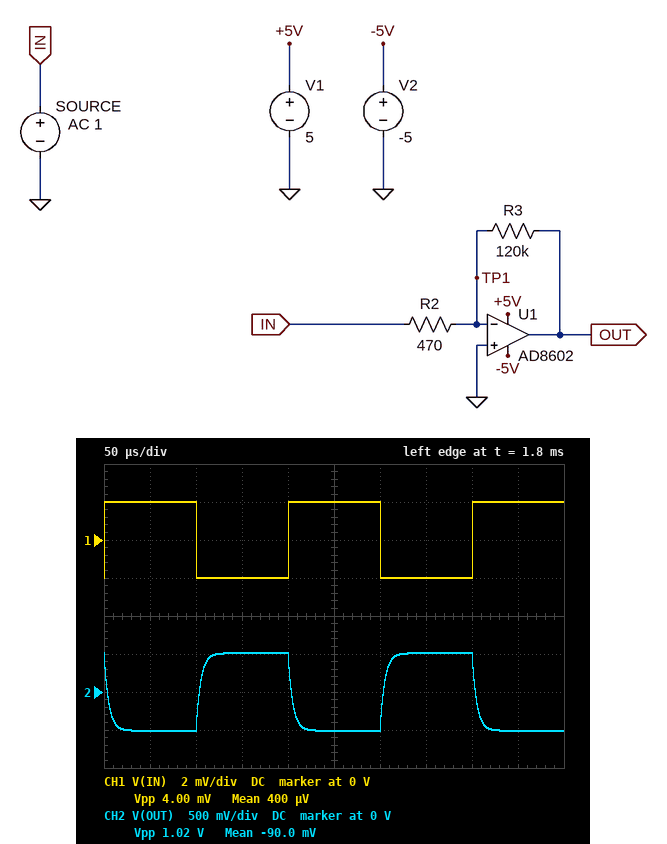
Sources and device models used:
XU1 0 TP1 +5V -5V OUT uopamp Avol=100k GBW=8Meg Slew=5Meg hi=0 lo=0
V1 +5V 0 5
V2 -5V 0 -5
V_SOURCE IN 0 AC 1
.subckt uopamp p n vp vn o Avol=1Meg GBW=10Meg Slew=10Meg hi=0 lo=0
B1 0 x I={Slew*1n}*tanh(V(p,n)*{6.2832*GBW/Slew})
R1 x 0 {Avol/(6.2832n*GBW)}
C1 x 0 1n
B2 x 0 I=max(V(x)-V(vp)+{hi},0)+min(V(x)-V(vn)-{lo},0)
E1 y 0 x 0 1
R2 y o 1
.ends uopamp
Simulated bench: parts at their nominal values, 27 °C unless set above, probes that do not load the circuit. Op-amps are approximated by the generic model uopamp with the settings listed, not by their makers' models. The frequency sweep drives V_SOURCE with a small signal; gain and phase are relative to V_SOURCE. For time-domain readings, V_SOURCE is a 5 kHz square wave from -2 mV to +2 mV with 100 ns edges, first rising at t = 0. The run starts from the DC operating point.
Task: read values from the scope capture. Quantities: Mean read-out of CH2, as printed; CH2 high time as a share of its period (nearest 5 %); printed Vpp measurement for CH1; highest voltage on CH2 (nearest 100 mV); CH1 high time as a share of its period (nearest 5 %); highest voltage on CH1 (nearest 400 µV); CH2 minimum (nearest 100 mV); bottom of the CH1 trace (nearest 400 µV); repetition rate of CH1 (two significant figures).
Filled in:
-90.0 mV
50 %
4.00 mV
500 mV
50 %
2.0 mV
-500 mV
-2.0 mV
5.0 kHz
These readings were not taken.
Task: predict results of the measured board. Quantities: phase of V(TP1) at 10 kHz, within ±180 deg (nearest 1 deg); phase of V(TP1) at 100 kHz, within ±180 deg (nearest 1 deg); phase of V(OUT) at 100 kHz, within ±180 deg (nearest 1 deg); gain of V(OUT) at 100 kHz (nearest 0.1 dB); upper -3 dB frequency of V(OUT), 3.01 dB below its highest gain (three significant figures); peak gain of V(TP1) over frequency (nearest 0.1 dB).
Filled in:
72 deg
17 deg
107 deg
37.6 dB
31.3 kHz
0 dB
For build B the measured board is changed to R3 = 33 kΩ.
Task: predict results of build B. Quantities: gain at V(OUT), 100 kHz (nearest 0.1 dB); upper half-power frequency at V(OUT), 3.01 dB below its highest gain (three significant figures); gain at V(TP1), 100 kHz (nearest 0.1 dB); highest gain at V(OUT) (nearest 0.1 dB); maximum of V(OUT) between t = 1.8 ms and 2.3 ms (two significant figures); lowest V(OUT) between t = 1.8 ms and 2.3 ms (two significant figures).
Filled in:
34.4 dB
112 kHz
-3.7 dB
36.9 dB
140 mV
-140 mV
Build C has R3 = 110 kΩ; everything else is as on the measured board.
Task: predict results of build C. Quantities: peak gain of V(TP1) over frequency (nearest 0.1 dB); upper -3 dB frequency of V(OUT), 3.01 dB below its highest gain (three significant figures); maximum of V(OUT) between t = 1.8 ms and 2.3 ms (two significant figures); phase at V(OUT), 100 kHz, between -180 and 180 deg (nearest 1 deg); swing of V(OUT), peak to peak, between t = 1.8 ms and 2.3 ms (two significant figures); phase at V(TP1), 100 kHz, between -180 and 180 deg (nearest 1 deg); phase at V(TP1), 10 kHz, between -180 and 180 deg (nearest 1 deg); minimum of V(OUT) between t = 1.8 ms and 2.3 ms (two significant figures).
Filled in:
0 dB
34.1 kHz
470 mV
109 deg
930 mV
19 deg
73 deg
-470 mV
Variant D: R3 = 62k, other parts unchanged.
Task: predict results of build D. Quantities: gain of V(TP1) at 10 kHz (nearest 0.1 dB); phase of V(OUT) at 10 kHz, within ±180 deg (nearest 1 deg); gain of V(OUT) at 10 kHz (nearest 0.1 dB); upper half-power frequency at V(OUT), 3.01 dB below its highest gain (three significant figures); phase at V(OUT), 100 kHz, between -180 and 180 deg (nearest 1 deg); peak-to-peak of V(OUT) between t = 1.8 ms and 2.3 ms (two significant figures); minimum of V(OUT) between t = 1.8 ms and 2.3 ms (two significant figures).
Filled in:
-15.8 dB
171 deg
42.3 dB
60.3 kHz
121 deg
530 mV
-260 mV
